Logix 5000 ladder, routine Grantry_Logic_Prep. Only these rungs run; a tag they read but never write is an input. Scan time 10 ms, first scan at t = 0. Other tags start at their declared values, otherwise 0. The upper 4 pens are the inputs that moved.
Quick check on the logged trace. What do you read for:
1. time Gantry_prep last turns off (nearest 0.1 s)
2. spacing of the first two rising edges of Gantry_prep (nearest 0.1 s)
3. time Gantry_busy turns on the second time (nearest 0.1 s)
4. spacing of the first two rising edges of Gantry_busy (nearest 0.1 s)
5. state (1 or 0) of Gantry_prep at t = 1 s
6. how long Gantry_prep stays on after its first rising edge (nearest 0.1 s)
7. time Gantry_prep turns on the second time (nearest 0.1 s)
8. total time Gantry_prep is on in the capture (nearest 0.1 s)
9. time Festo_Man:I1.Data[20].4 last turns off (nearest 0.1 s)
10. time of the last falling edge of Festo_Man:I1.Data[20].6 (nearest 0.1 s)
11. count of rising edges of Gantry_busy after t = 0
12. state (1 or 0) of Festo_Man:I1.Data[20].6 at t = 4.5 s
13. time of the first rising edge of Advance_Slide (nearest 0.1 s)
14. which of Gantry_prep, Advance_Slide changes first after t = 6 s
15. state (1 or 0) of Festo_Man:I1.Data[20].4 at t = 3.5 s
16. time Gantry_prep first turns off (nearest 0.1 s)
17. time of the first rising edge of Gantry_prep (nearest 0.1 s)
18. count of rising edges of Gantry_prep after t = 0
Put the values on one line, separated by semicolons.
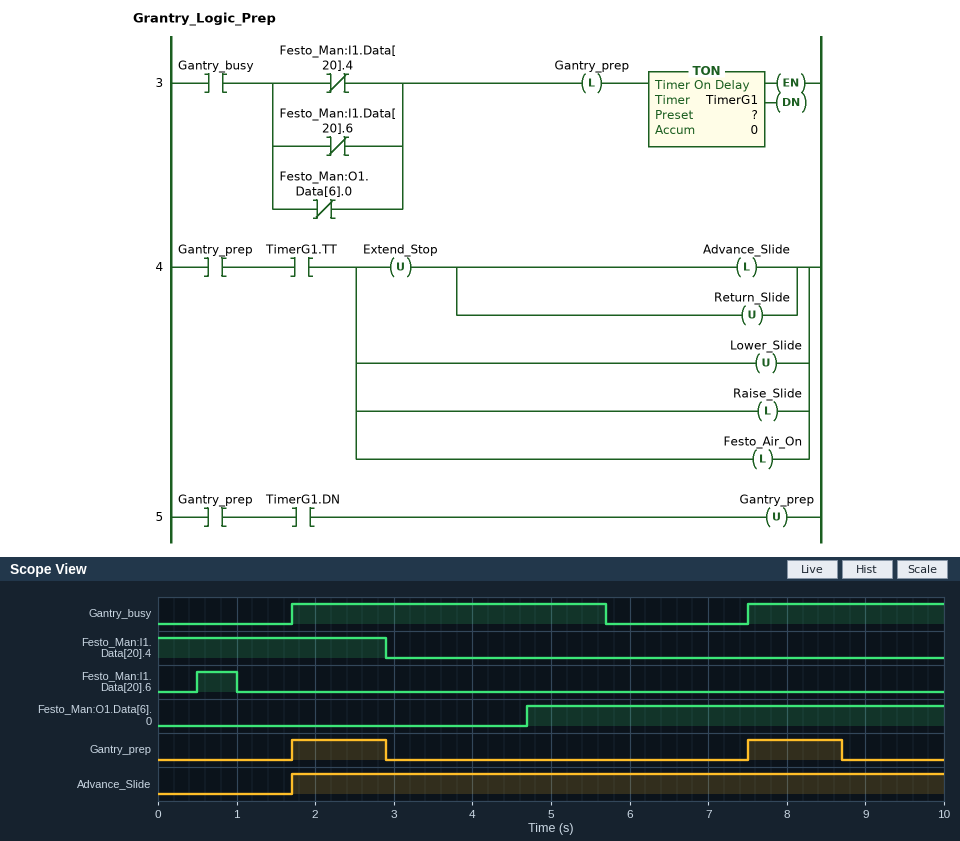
8.7 s; 5.8 s; 7.5 s; 5.8 s; 0; 1.2 s; 7.5 s; 2.4 s; 2.9 s; 1.0 s; 2; 0; 1.7 s; Gantry_prep; 0; 2.9 s; 1.7 s; 2
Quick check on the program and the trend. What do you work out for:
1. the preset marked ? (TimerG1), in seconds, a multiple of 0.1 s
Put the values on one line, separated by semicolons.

1.2 s
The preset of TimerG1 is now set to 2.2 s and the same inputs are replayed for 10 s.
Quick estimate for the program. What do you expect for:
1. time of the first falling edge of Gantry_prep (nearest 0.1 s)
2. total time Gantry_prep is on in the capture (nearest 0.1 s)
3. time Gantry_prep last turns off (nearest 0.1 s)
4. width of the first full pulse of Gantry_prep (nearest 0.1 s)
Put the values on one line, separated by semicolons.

3.9 s; 4.4 s; 9.7 s; 2.2 s
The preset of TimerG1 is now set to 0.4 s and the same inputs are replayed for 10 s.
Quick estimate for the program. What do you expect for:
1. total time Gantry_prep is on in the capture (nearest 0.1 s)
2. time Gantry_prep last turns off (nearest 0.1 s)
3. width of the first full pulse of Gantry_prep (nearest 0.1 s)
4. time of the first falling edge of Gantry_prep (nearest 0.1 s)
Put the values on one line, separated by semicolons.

0.8 s; 7.9 s; 0.4 s; 2.1 s
